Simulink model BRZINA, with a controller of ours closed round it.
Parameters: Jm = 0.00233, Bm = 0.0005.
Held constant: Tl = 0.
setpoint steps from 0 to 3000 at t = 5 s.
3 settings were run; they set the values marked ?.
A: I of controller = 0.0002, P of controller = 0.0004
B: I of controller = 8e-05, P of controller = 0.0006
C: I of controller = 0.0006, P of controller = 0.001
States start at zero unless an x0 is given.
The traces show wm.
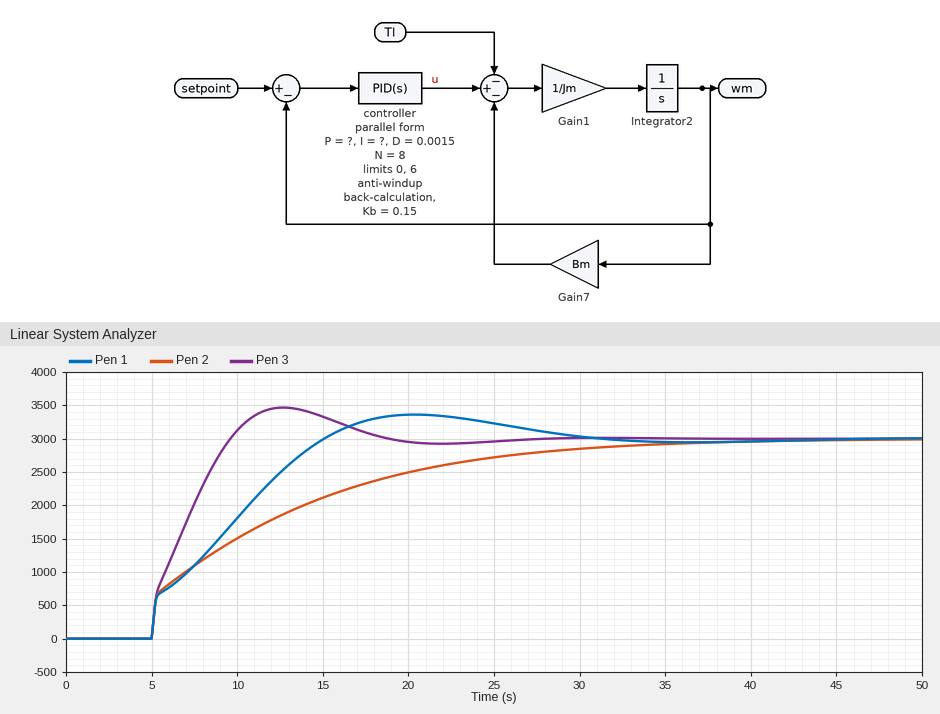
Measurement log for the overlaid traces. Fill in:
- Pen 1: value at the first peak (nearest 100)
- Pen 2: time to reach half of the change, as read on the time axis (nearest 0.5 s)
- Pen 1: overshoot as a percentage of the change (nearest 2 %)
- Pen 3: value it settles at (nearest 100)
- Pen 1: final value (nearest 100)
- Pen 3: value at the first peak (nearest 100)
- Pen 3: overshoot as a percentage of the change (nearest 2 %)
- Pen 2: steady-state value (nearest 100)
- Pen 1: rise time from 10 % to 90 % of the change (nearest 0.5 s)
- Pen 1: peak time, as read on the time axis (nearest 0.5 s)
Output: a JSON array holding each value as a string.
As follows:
["3400", "10.0 s", "12 %", "3000", "3000", "3500", "16 %", "3000", "8.5 s", "20.5 s"]
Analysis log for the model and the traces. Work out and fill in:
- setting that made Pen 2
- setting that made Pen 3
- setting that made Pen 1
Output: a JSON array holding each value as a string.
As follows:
["B", "C", "A"]
